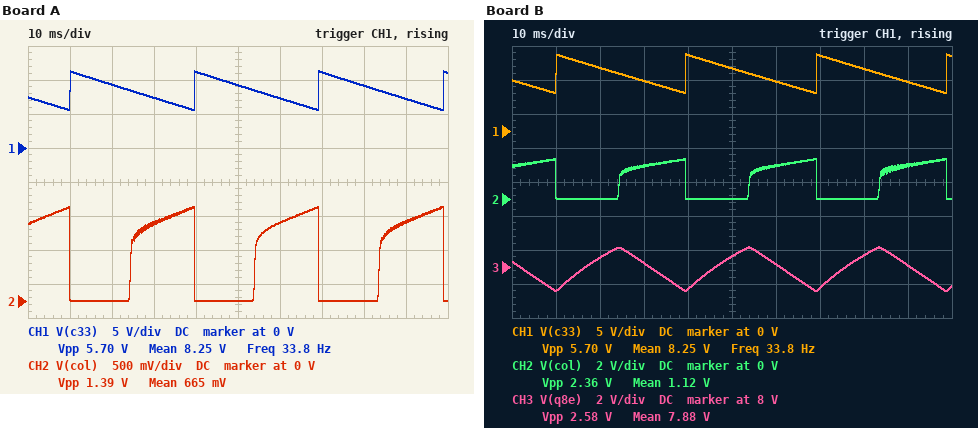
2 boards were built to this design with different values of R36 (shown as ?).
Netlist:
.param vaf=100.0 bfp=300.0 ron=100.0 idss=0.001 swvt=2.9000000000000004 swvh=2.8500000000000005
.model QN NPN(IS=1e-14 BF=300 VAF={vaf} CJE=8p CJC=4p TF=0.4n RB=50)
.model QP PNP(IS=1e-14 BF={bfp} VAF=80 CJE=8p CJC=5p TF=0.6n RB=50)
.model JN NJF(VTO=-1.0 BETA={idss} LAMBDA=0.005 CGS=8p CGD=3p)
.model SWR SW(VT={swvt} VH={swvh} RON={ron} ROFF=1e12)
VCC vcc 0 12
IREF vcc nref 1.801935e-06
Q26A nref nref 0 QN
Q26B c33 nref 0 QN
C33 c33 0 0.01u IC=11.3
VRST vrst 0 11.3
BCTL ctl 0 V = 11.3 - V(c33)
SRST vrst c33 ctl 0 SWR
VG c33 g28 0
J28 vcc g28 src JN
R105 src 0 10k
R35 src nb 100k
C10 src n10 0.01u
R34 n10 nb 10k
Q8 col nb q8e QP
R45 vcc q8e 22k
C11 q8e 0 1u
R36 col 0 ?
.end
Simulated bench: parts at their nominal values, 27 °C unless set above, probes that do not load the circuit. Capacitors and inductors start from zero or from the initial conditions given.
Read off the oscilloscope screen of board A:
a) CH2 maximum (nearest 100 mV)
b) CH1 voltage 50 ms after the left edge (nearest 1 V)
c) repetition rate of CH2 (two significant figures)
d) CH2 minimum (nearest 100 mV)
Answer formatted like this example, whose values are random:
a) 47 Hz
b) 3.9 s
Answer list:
a) 1.4 V
b) 9 V
c) 34 Hz
d) 0 V
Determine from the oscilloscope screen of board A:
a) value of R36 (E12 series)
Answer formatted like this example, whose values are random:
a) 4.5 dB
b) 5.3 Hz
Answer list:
a) 3.3 kΩ
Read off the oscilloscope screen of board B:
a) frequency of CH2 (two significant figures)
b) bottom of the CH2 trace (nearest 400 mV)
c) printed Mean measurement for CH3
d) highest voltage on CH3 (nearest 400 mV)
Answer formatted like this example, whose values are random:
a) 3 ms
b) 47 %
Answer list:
a) 34 Hz
b) 0 V
c) 7.88 V
d) 9.2 V
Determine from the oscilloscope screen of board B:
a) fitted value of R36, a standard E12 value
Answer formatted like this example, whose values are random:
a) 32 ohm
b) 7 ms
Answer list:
a) 5.6 kΩ
